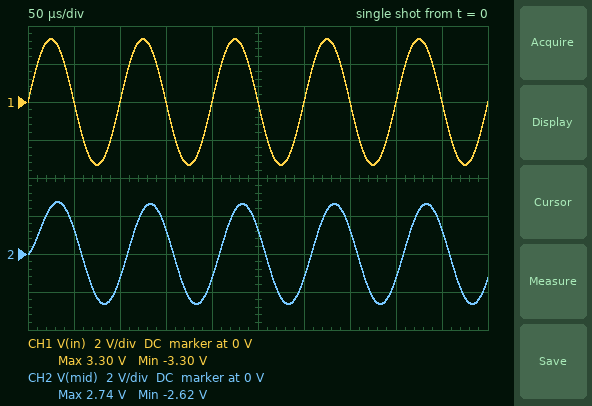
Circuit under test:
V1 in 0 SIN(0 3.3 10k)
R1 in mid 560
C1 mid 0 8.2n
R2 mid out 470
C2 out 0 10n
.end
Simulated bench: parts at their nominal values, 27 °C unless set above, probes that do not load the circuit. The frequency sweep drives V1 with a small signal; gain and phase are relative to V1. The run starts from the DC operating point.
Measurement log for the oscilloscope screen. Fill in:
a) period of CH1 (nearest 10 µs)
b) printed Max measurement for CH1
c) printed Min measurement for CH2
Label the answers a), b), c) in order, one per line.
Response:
a) 100 µs
b) 3.30 V
c) -2.62 V
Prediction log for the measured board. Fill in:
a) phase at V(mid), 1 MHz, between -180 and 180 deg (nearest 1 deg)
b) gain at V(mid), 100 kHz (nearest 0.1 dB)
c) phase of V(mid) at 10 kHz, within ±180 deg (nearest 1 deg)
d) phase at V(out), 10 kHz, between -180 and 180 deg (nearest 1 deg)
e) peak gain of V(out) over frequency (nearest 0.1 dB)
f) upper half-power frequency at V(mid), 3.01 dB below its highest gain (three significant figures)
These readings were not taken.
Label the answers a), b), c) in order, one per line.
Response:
a) -86 deg
b) -11.7 dB
c) -29 deg
d) -46 deg
e) 0 dB
f) 13.6 kHz
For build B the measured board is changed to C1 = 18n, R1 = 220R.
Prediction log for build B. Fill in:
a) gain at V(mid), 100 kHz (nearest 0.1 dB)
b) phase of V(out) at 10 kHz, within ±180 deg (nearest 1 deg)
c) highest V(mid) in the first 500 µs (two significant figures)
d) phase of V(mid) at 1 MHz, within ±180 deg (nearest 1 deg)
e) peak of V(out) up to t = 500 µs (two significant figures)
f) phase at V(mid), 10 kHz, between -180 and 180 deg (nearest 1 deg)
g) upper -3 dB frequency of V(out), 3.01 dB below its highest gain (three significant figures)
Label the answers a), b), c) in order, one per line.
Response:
a) -9.5 dB
b) -36 deg
c) 3.0 V
d) -87 deg
e) 2.9 V
f) -20 deg
g) 17.3 kHz
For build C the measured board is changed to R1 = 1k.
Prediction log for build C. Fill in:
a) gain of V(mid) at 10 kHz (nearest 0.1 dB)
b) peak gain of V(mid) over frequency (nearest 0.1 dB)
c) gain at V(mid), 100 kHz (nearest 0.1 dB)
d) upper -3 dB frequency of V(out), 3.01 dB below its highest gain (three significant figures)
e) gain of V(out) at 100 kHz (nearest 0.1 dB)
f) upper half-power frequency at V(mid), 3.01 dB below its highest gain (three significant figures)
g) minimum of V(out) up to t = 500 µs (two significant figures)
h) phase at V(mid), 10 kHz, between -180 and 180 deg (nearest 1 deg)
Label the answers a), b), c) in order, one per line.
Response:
a) -4.1 dB
b) 0 dB
c) -16.2 dB
d) 7.50 kHz
e) -26.1 dB
f) 7.89 kHz
g) -2.0 V
h) -43 deg
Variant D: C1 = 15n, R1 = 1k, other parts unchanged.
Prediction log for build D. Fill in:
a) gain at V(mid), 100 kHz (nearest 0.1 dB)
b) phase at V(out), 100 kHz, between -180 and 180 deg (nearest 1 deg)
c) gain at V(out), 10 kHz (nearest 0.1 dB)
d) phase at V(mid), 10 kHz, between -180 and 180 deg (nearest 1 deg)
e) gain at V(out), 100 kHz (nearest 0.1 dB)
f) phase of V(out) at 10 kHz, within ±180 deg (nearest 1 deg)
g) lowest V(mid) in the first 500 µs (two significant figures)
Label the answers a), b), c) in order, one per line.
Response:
a) -20.4 dB
b) -145 deg
c) -6.0 dB
d) -52 deg
e) -30.3 dB
f) -69 deg
g) -1.7 V
